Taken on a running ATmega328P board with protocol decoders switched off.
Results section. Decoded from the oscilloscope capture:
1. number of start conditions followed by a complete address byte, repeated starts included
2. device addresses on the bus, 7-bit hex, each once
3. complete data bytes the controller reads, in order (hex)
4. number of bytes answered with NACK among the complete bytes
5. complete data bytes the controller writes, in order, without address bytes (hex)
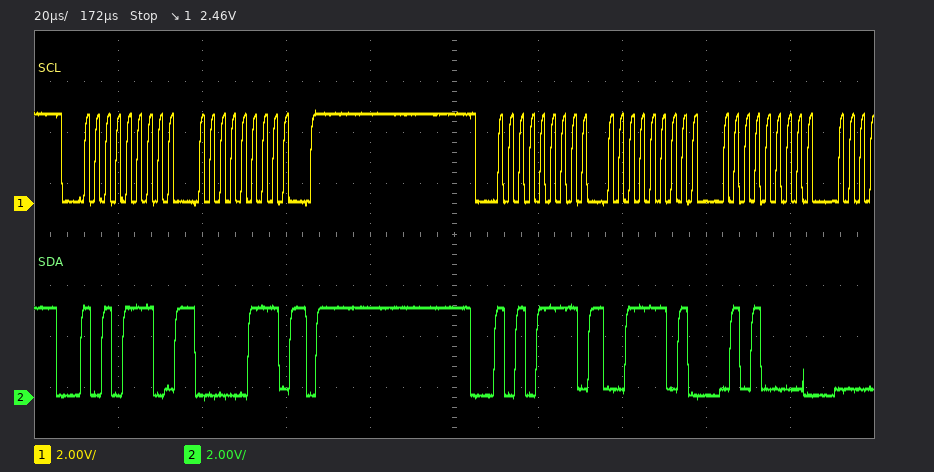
2
0x57
3D 50
0
07
